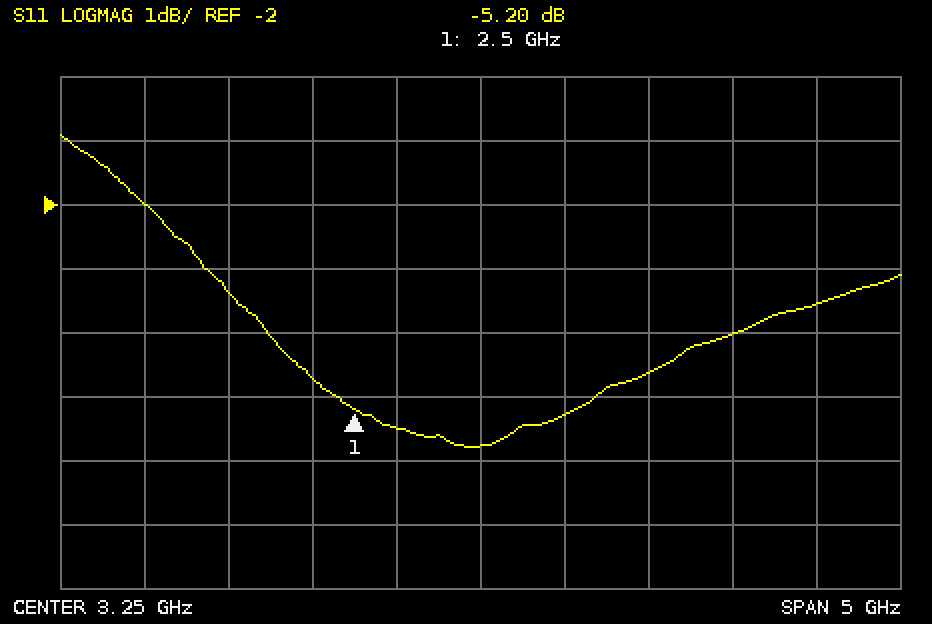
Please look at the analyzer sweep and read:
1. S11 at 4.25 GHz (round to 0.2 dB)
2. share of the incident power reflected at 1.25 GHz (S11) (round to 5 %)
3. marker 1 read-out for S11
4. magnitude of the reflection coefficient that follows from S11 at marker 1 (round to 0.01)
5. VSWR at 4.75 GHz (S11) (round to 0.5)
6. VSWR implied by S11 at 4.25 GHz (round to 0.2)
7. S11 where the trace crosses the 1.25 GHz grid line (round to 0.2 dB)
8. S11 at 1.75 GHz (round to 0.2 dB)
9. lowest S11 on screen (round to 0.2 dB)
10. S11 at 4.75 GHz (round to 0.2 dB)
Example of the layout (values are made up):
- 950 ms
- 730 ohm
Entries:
- -4.6 dB
- 65 %
- -5.20 dB
- 0.55
- 4.5
- 3.8
- -2.0 dB
- -3.4 dB
- -5.8 dB
- -4.0 dB
